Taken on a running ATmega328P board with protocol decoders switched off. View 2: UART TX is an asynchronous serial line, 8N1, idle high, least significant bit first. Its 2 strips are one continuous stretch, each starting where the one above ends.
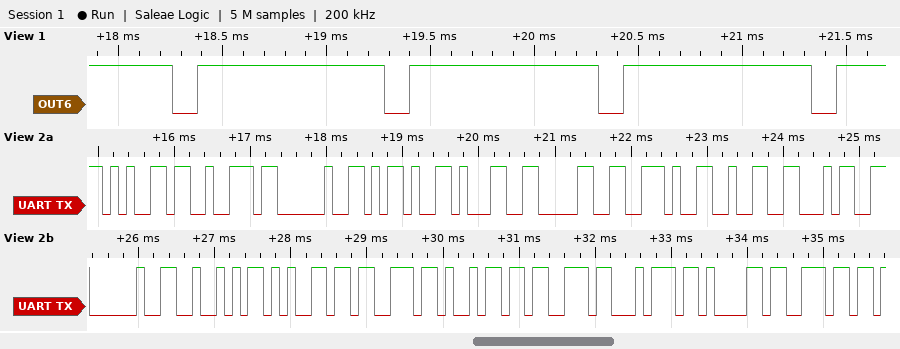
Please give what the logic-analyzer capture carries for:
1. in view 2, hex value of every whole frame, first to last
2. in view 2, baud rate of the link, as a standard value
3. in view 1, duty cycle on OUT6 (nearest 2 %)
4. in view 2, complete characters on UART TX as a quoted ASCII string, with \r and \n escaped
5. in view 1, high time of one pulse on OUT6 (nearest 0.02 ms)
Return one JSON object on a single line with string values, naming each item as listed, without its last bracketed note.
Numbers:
{"in view 2, hex value of every whole frame, first to last": "0x65 0x72 0x20 0x2D 0x31 0x30 0x2E 0x32 0x34 0x20 0x52 0x65 0x73 0x69 0x73 0x74 0x61 0x6E", "in view 2, baud rate of the link, as a standard value": "9600 baud", "in view 1, duty cycle on OUT6": "88 %", "in view 2, complete characters on UART TX as a quoted ASCII string, with \\r and \\n escaped": "\"er -10.24 Resistan\"", "in view 1, high time of one pulse on OUT6": "0.90 ms"}
